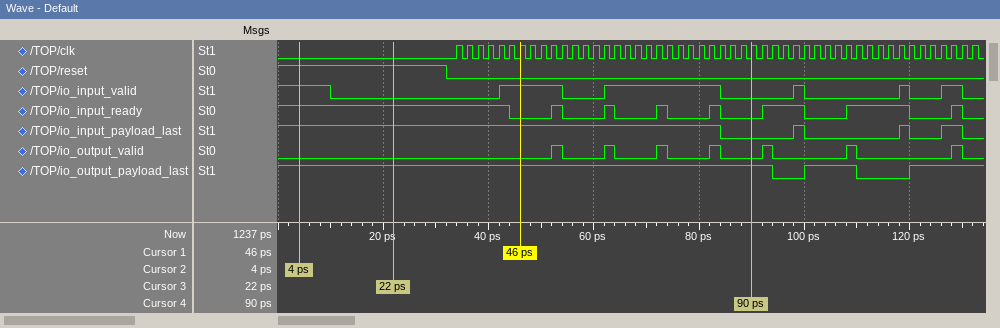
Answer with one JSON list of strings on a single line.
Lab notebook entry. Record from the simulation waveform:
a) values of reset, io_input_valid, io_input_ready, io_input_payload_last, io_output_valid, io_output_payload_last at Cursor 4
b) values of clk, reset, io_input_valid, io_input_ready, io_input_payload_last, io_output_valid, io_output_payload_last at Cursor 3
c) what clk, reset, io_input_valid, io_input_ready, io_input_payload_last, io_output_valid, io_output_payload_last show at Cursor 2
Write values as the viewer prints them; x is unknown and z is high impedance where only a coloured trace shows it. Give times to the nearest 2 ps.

["reset=0, io_input_valid=0, io_input_ready=0, io_input_payload_last=0, io_output_valid=0, io_output_payload_last=1", "clk=0, reset=1, io_input_valid=0, io_input_ready=1, io_input_payload_last=1, io_output_valid=0, io_output_payload_last=1", "clk=0, reset=1, io_input_valid=1, io_input_ready=1, io_input_payload_last=1, io_output_valid=0, io_output_payload_last=1"]
